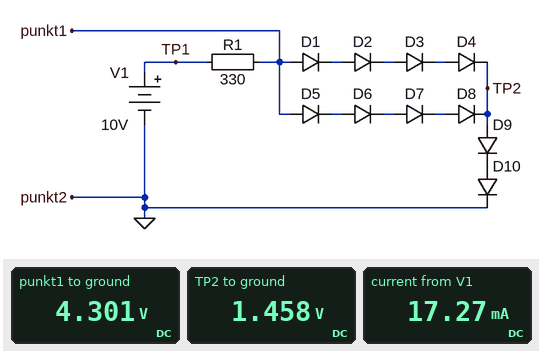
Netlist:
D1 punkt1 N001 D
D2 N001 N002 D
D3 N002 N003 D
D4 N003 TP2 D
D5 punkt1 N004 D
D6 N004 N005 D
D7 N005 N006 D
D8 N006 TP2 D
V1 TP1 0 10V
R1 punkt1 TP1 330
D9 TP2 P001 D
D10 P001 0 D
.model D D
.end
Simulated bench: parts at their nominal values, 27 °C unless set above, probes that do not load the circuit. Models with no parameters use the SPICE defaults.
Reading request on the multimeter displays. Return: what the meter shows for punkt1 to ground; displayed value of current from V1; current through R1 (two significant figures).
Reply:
4.301 V
17.27 mA
17 mA
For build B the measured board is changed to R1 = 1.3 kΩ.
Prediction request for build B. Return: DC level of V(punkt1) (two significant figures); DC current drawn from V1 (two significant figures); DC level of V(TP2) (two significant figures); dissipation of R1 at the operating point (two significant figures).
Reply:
4.1 V
4.5 mA
1.4 V
27 mW
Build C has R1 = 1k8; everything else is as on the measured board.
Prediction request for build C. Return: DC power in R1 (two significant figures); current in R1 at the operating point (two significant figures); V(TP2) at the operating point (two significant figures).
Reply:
20 mW
3.3 mA
1.4 V
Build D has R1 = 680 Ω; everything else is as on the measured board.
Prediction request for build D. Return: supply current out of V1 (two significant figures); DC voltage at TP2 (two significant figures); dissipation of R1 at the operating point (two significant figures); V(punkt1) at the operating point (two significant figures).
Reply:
8.5 mA
1.4 V
50 mW
4.2 V
